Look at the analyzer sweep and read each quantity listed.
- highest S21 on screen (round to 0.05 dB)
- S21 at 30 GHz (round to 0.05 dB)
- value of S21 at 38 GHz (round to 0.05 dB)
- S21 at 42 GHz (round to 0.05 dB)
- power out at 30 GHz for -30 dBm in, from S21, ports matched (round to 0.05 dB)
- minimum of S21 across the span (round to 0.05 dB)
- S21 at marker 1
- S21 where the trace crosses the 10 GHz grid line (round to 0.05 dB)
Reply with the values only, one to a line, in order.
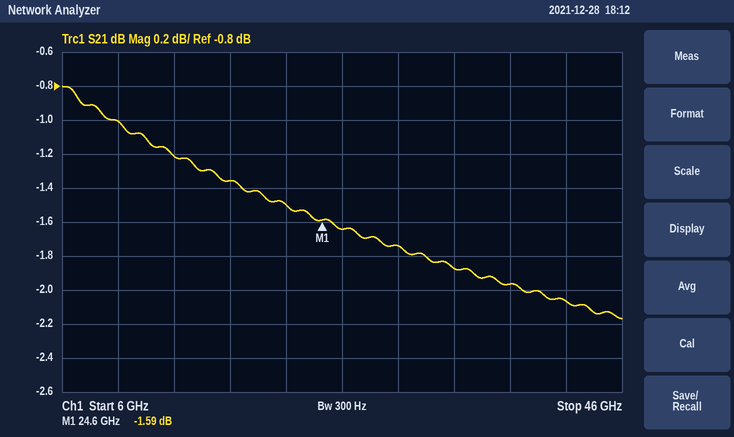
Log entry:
-0.80 dB
-1.75 dB
-1.95 dB
-2.05 dB
-31.75 dBm
-2.15 dB
-1.59 dB
-1.00 dB
